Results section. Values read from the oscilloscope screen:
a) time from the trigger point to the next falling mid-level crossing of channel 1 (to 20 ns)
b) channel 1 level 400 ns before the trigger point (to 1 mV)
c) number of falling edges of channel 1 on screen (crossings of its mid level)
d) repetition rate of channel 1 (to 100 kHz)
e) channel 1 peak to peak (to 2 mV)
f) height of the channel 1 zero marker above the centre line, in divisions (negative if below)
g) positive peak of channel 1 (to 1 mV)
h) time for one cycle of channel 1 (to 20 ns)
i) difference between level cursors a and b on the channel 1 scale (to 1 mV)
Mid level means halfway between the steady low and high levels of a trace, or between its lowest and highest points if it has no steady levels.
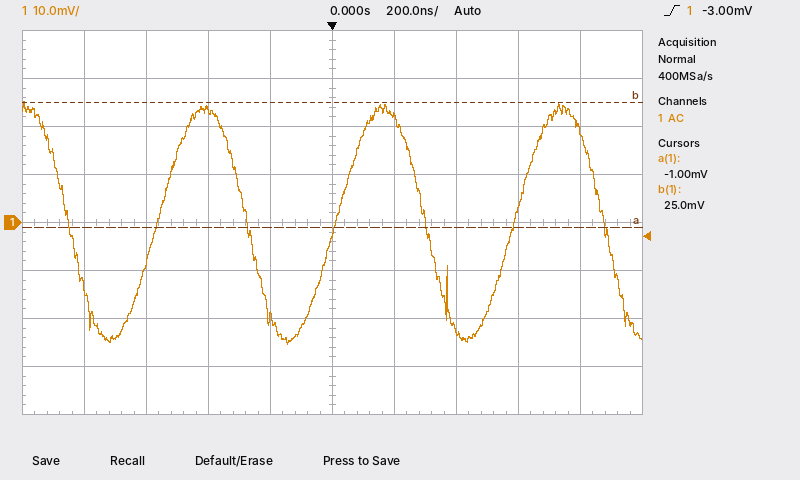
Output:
300 ns
23 mV
4
1.7 MHz
50 mV
0.0 div
25 mV
580 ns
26 mV
